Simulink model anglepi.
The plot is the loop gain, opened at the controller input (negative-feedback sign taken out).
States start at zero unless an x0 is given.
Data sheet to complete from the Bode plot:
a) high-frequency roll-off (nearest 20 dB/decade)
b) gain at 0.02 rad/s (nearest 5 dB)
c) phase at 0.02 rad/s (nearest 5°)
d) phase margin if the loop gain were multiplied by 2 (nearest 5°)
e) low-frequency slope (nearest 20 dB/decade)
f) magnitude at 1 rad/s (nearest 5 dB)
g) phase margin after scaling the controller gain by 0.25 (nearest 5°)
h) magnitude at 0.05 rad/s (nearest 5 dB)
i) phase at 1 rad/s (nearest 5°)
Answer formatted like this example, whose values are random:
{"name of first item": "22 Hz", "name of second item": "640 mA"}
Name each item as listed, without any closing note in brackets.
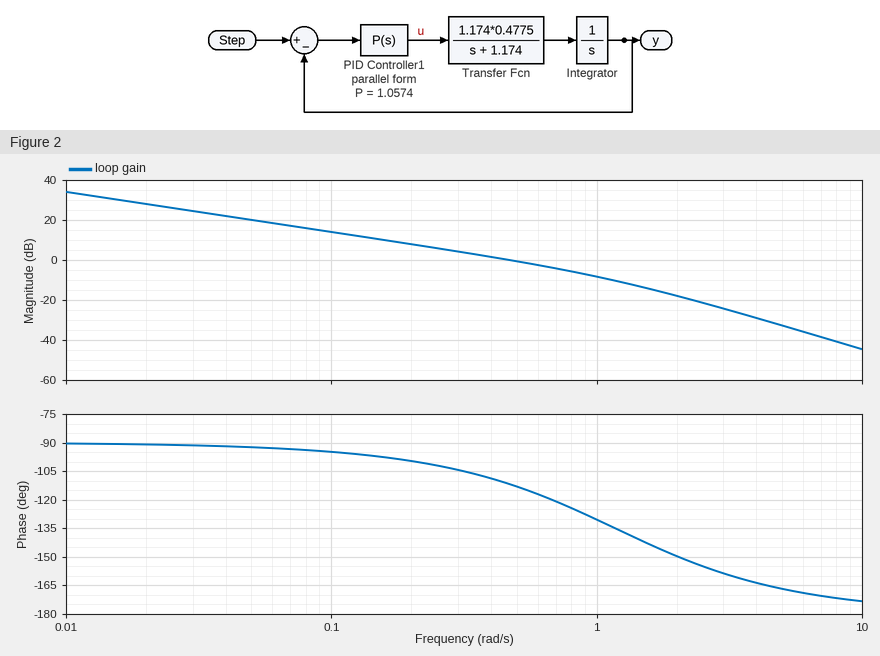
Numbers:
{"high-frequency roll-off": "-40 dB/decade", "gain at 0.02 rad/s": "30 dB", "phase at 0.02 rad/s": "-90°", "phase margin if the loop gain were multiplied by 2": "55°", "low-frequency slope": "-20 dB/decade", "magnitude at 1 rad/s": "-10 dB", "phase margin after scaling the controller gain by 0.25": "85°", "magnitude at 0.05 rad/s": "20 dB", "phase at 1 rad/s": "-130°"}
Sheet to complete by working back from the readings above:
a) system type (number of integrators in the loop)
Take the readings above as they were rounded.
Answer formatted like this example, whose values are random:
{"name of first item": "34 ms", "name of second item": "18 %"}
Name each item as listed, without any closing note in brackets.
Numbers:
{"system type": "1"}
